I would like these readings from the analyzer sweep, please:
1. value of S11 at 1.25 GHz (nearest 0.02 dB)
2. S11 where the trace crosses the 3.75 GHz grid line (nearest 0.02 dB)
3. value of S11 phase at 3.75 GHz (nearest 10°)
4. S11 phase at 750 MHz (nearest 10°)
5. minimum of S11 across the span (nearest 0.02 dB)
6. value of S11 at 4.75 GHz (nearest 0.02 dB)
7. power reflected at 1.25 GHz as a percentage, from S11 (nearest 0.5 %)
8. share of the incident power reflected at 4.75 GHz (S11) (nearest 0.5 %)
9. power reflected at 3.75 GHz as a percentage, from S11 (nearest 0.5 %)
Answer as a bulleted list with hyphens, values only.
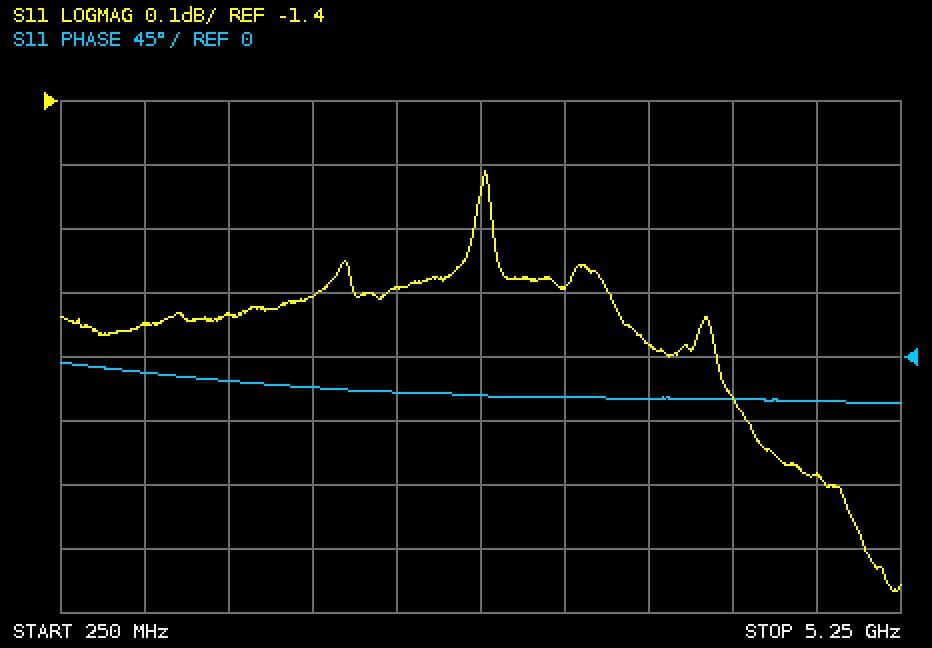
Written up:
- -1.74 dB
- -1.78 dB
- -30°
- -10°
- -2.16 dB
- -1.98 dB
- 67.0 %
- 63.5 %
- 66.5 %
